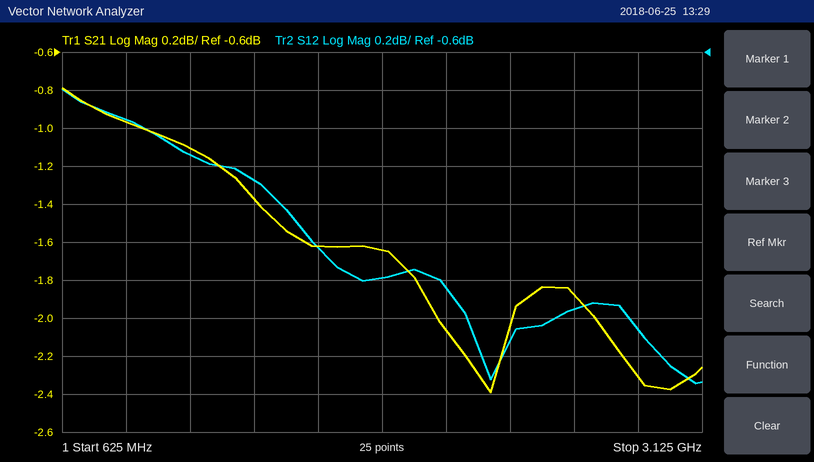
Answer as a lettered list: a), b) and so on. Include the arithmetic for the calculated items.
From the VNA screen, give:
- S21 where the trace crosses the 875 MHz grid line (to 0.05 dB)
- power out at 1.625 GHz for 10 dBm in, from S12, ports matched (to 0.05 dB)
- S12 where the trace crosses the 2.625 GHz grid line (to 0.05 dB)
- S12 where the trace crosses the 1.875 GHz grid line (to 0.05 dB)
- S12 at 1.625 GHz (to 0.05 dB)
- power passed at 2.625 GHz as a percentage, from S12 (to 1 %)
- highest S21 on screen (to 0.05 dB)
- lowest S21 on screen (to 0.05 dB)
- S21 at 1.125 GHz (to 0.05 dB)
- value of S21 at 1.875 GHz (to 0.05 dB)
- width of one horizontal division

a) -0.95 dB
b) 10 dBm + (-1.65 dB) = 8.35 dBm
c) -1.95 dB
d) -1.80 dB
e) -1.65 dB
f) 10^(-1.95/10) ≈ 64 %
g) -0.80 dB
h) -2.40 dB
i) -1.10 dB
j) -1.65 dB
k) 250 MHz
